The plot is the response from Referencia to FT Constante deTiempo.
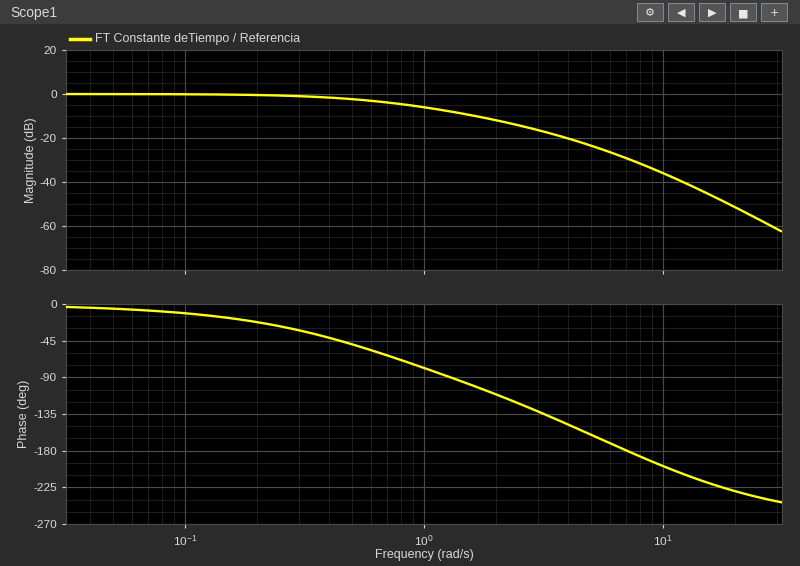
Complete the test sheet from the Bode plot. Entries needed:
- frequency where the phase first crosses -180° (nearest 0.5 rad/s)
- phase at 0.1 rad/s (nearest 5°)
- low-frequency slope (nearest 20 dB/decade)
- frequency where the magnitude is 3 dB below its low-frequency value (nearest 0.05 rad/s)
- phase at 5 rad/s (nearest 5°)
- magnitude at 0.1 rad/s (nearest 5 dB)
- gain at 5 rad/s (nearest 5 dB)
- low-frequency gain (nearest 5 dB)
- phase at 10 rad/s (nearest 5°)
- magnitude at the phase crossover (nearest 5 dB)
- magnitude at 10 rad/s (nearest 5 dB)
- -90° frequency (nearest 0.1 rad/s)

7.0 rad/s
-10°
0 dB/decade
0.60 rad/s
-160°
0 dB
-25 dB
0 dB
-200°
-30 dB
-35 dB
1.3 rad/s
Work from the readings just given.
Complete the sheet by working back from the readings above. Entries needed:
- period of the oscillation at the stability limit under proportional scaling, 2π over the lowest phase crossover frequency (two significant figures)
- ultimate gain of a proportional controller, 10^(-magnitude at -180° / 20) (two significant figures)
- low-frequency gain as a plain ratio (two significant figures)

0.90 s
32
1.0
